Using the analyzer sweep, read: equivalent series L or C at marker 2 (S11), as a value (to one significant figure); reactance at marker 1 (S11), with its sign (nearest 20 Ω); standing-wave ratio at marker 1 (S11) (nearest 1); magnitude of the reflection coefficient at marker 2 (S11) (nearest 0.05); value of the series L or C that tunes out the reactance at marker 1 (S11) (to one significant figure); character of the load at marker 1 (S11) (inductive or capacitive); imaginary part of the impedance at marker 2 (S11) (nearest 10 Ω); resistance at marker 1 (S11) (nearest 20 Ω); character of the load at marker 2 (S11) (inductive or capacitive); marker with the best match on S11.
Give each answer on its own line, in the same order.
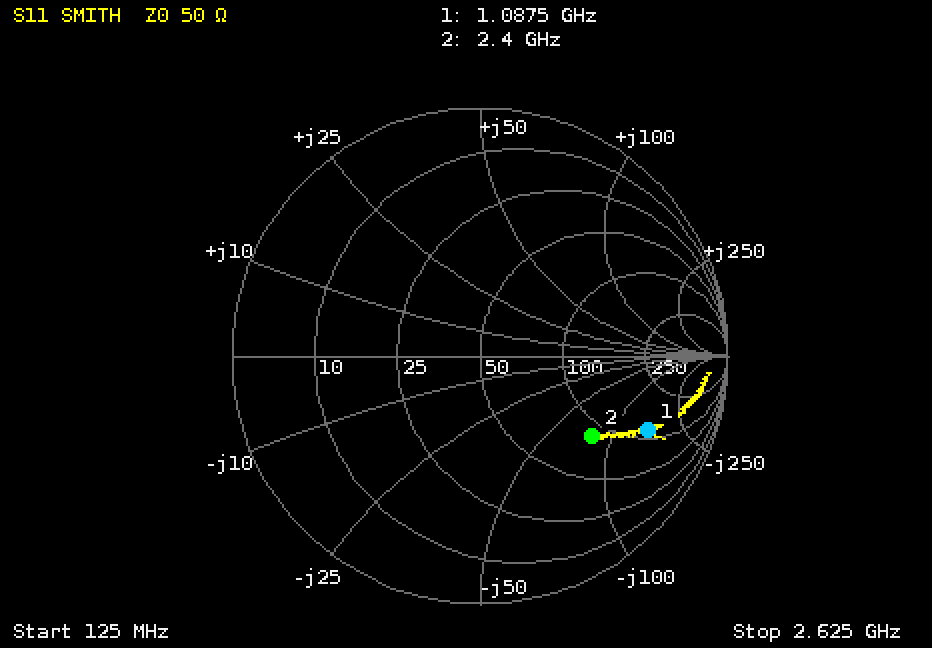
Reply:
800 fF
-160 Ω
7
0.55
20 nH
capacitive
-80 Ω
120 Ω
capacitive
marker 2
